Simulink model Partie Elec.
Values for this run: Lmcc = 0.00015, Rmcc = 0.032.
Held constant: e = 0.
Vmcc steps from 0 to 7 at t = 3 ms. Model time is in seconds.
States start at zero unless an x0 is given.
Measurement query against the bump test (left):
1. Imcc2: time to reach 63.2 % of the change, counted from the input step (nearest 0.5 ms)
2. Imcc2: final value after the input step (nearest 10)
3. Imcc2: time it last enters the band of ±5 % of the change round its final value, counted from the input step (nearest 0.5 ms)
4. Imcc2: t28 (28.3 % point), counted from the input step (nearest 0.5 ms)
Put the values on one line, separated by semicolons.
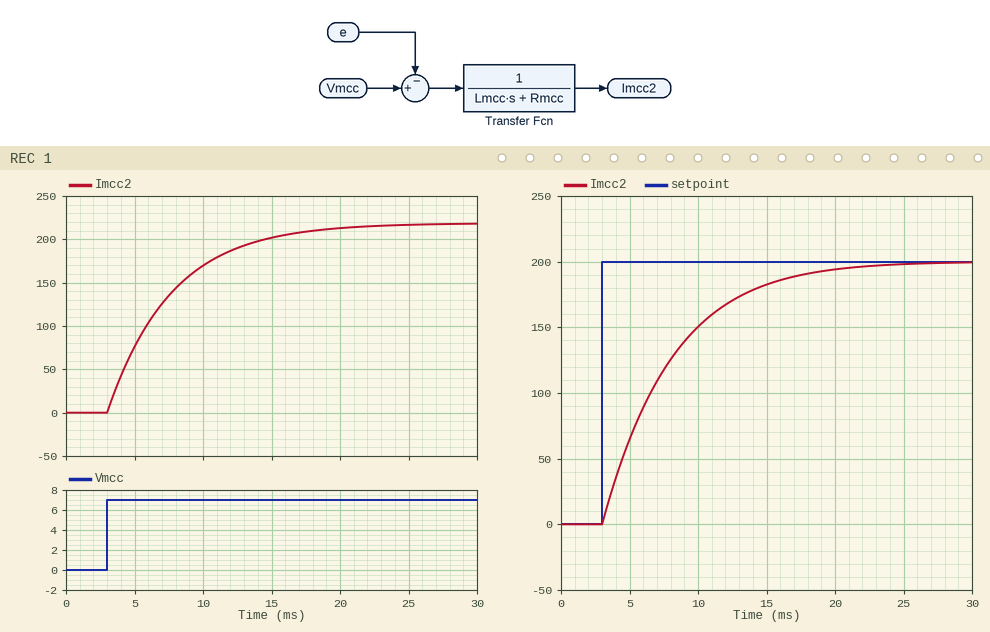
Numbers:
4.5 ms; 220; 14.0 ms; 1.5 ms
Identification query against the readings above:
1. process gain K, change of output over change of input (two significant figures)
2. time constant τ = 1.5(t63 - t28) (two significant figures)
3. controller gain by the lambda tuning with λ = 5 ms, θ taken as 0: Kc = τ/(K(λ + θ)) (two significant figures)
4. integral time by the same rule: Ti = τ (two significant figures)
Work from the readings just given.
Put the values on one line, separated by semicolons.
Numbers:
31; 4.5 ms; 0.029; 4.5 ms
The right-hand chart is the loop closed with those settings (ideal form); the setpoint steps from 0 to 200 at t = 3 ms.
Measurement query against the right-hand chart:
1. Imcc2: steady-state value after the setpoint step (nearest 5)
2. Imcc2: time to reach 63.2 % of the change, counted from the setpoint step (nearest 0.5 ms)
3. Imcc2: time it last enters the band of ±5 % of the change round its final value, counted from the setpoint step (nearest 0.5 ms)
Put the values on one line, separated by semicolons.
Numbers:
200; 5.0 ms; 14.5 ms
